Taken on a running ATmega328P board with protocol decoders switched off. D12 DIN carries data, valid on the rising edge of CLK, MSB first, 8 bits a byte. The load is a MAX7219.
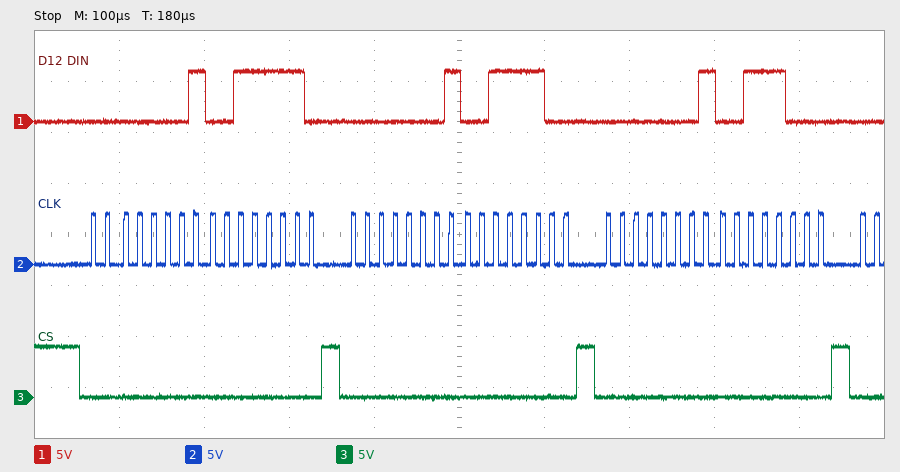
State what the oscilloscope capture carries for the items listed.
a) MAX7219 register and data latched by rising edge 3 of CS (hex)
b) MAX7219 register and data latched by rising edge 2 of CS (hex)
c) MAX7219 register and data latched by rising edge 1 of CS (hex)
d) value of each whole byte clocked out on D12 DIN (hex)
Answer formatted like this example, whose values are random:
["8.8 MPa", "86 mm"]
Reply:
["register 0x1, data 0x38", "register 0x1, data 0x3C", "register 0x1, data 0x3E", "0x01 0x3E 0x01 0x3C 0x01 0x38"]
